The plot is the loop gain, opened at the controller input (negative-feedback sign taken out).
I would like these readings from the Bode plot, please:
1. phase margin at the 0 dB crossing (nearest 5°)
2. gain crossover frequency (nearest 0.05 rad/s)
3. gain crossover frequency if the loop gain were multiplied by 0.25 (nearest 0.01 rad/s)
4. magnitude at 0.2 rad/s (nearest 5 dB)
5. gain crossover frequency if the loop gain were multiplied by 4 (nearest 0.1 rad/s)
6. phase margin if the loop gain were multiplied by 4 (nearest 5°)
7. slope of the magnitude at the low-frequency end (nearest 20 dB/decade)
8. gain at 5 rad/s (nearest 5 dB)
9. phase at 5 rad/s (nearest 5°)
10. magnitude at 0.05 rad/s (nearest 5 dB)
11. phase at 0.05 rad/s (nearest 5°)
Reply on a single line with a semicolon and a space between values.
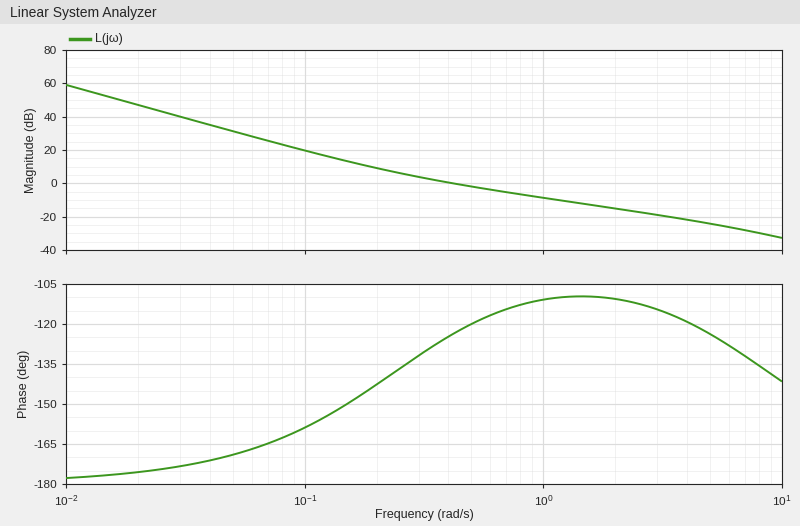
55°; 0.40 rad/s; 0.16 rad/s; 10 dB; 1.4 rad/s; 70°; -40 dB/decade; -25 dB; -125°; 30 dB; -170°
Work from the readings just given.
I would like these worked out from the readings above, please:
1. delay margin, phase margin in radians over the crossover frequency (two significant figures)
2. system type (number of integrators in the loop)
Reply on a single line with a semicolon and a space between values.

2.4 s; 2
